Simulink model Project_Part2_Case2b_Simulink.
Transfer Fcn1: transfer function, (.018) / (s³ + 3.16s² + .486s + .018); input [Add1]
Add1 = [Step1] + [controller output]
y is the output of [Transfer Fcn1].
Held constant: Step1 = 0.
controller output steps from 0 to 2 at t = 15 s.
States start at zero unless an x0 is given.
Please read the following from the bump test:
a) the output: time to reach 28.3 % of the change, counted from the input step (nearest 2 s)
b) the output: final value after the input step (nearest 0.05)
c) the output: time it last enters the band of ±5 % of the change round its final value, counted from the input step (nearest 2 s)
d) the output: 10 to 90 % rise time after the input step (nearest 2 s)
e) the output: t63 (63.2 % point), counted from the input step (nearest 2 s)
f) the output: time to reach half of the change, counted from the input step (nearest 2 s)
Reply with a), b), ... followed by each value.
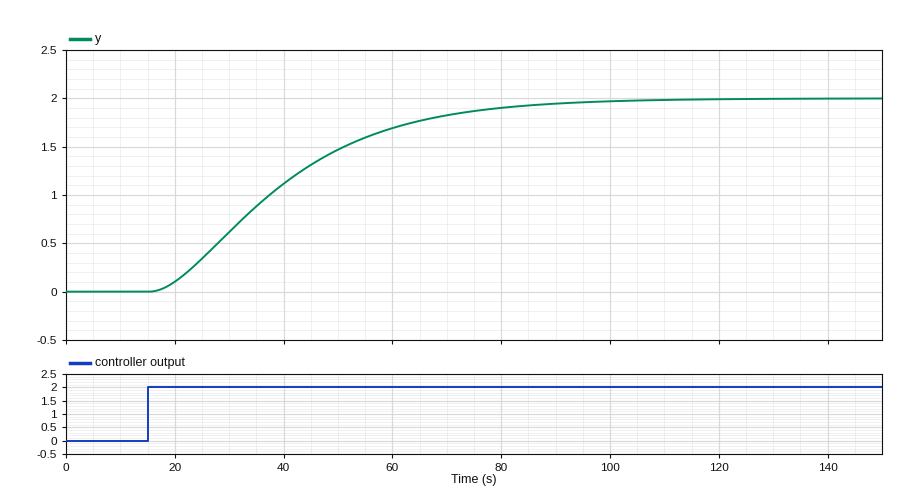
a) 14 s
b) 2.00
c) 64 s
d) 46 s
e) 28 s
f) 22 s
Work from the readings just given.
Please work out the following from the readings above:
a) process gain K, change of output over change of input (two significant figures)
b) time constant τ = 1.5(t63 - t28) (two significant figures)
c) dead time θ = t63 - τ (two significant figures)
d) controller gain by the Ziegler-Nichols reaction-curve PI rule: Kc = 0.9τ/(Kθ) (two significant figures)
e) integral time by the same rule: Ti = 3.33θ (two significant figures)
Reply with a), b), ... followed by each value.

a) 1.0
b) 21 s
c) 7.0 s
d) 2.7
e) 23 s
